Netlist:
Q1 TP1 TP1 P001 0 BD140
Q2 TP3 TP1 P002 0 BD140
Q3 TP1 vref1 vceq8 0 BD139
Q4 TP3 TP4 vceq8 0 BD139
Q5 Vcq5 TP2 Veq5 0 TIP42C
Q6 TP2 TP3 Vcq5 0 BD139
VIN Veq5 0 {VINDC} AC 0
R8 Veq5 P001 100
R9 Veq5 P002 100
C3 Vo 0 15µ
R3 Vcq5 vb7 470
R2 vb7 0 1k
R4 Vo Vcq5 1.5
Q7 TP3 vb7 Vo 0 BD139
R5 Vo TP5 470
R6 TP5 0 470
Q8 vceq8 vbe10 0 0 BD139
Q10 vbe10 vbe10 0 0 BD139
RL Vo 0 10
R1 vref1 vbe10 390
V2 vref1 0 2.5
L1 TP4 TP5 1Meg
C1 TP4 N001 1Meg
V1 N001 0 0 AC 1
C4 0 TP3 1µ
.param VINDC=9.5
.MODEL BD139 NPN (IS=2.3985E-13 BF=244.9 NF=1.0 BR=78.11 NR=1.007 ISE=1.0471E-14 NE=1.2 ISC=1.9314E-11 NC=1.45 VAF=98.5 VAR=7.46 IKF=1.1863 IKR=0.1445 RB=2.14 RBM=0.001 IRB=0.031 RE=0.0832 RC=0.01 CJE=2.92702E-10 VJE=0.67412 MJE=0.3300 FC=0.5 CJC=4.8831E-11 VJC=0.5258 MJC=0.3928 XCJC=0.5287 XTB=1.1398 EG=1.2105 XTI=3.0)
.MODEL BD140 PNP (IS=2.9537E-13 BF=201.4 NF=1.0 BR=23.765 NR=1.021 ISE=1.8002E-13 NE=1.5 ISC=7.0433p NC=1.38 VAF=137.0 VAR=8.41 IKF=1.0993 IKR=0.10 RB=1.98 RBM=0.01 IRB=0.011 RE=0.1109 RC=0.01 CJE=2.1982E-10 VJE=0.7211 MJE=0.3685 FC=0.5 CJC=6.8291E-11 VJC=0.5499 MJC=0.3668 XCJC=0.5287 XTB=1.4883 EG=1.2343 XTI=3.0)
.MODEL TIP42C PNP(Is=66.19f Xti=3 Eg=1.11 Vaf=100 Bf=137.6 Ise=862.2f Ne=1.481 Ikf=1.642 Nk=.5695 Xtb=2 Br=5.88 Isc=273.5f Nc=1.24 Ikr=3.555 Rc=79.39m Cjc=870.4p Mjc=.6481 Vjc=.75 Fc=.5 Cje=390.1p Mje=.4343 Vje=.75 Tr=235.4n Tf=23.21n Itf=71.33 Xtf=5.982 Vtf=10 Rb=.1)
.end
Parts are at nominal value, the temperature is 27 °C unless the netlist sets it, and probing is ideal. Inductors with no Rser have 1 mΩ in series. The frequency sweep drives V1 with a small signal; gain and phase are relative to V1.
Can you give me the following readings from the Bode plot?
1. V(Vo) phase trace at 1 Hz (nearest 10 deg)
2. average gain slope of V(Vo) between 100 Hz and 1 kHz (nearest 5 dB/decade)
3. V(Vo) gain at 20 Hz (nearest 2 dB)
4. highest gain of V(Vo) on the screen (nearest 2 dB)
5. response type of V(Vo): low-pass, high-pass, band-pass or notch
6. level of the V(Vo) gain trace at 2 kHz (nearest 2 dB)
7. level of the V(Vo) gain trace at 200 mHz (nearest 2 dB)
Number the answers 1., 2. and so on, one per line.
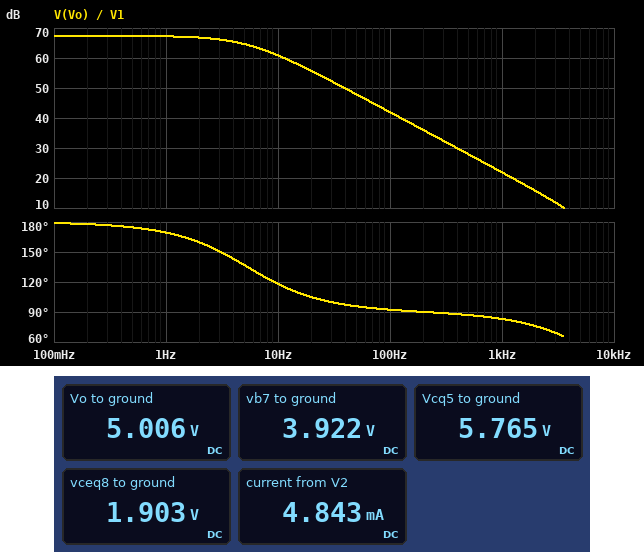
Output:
1. 170 deg
2. -20 dB/decade
3. 56 dB
4. 68 dB
5. low-pass
6. 16 dB
7. 68 dB
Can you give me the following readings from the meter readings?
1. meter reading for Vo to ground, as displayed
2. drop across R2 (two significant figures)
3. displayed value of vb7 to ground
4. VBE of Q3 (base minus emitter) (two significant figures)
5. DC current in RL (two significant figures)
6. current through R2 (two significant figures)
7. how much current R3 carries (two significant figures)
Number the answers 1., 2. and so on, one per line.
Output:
1. 5.006 V
2. 3.9 V
3. 3.922 V
4. 600 mV
5. 500 mA
6. 3.9 mA
7. 3.9 mA
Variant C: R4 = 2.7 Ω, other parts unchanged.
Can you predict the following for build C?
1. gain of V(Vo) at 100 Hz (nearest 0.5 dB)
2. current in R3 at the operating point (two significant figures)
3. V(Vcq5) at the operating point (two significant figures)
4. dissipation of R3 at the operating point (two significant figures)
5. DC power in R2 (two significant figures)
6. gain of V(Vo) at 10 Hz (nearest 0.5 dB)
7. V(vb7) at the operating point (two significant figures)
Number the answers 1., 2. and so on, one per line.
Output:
1. 41.0 dB
2. 4.3 mA
3. 6.4 V
4. 8.8 mW
5. 19 mW
6. 60.0 dB
7. 4.3 V
